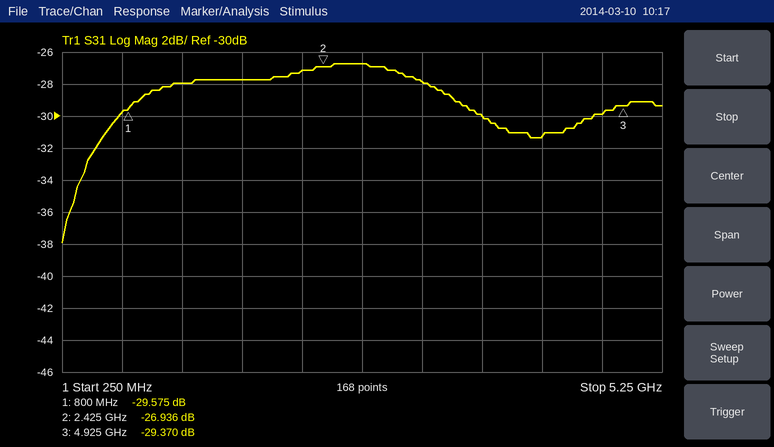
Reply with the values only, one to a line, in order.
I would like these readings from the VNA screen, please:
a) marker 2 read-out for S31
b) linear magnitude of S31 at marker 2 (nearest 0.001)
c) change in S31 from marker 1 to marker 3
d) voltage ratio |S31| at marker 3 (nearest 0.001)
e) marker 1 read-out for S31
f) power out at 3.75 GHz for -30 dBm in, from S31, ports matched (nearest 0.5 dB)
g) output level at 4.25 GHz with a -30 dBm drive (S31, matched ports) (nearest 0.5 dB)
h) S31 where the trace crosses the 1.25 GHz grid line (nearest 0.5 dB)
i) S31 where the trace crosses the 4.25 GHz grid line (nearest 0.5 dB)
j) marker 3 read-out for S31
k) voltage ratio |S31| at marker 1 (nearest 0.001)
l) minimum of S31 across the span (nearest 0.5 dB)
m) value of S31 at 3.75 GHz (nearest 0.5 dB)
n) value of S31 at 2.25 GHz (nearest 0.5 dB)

-26.936 dB
0.045
0.205 dB
0.034
-29.575 dB
-60.0 dBm
-61.5 dBm
-28.0 dB
-31.5 dB
-29.370 dB
0.033
-38.0 dB
-30.0 dB
-27.0 dB
